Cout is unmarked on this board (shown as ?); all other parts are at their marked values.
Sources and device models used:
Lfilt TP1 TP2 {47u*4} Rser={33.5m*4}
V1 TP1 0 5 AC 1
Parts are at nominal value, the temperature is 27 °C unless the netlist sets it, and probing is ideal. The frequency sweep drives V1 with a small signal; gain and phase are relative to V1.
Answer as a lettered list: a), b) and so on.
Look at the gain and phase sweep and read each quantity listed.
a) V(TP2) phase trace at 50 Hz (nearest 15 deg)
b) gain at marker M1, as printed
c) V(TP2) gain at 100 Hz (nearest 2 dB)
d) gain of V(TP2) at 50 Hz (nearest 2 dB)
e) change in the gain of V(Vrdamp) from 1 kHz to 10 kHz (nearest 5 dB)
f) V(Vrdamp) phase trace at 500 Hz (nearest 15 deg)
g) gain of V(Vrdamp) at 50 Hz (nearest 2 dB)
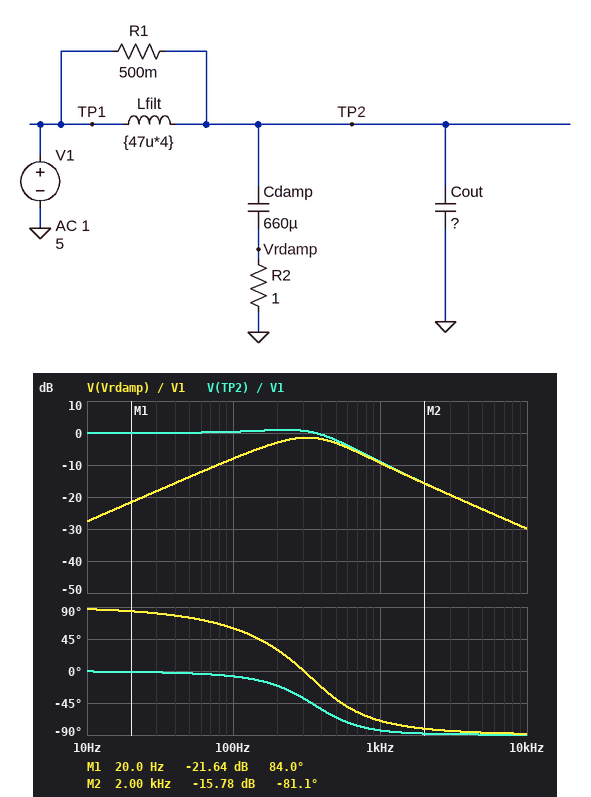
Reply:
a) 0 deg
b) -21.64 dB
c) 0 dB
d) 0 dB
e) -20 dB
f) -45 deg
g) -14 dB
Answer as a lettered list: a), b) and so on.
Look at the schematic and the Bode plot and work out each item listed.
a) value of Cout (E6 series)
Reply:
a) 1 mF
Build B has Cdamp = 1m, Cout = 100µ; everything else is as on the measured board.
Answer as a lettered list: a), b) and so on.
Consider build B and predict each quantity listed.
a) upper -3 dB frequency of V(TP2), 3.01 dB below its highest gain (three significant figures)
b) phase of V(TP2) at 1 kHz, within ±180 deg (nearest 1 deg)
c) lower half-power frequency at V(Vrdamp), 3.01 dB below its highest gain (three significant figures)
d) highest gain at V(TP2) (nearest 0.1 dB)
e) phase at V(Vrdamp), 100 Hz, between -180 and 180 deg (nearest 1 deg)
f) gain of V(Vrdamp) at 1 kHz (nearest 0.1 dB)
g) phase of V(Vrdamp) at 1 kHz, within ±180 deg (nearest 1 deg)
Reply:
a) 1.27 kHz
b) -21 deg
c) 113 Hz
d) 0 dB
e) 53 deg
f) -2.8 dB
g) -12 deg
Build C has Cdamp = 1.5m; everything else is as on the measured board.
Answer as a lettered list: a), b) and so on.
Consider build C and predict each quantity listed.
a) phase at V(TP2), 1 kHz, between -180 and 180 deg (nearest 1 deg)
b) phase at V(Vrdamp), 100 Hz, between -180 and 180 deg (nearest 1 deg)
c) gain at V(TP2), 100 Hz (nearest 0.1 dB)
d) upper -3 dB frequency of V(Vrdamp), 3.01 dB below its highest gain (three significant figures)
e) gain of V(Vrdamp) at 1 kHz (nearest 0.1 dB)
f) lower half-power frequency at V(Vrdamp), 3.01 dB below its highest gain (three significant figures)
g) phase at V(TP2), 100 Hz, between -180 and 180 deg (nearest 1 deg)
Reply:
a) -83 deg
b) 37 deg
c) 0.1 dB
d) 564 Hz
e) -9.0 dB
f) 94.1 Hz
g) -10 deg
